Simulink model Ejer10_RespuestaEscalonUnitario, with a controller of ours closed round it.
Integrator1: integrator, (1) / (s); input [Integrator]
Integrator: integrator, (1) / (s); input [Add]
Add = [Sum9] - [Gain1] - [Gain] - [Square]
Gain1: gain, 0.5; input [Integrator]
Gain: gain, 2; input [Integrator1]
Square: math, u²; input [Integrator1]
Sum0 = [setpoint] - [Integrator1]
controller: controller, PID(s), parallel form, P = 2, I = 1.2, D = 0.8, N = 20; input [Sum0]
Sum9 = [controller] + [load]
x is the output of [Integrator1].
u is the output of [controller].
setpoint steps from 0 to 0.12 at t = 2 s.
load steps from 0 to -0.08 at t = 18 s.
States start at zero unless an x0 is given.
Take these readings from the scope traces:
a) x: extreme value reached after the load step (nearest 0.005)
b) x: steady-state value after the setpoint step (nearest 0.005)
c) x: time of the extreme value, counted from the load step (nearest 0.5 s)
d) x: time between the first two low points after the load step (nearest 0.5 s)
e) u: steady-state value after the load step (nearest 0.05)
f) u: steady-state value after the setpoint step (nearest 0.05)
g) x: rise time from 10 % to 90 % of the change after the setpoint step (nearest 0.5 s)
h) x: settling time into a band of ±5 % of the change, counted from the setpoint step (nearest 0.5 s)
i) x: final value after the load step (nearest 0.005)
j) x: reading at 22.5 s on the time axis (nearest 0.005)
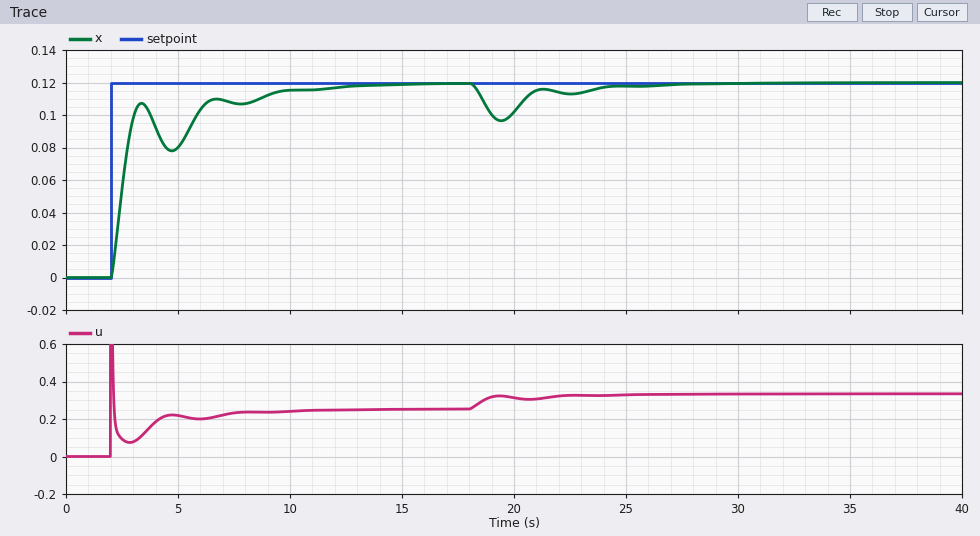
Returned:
0.095
0.120
1.5 s
3.0 s
0.35
0.25
4.0 s
7.5 s
0.120
0.115
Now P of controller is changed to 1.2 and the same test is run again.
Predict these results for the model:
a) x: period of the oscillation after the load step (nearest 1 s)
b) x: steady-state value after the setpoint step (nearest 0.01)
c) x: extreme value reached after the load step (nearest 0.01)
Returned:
4 s
0.12
0.09
